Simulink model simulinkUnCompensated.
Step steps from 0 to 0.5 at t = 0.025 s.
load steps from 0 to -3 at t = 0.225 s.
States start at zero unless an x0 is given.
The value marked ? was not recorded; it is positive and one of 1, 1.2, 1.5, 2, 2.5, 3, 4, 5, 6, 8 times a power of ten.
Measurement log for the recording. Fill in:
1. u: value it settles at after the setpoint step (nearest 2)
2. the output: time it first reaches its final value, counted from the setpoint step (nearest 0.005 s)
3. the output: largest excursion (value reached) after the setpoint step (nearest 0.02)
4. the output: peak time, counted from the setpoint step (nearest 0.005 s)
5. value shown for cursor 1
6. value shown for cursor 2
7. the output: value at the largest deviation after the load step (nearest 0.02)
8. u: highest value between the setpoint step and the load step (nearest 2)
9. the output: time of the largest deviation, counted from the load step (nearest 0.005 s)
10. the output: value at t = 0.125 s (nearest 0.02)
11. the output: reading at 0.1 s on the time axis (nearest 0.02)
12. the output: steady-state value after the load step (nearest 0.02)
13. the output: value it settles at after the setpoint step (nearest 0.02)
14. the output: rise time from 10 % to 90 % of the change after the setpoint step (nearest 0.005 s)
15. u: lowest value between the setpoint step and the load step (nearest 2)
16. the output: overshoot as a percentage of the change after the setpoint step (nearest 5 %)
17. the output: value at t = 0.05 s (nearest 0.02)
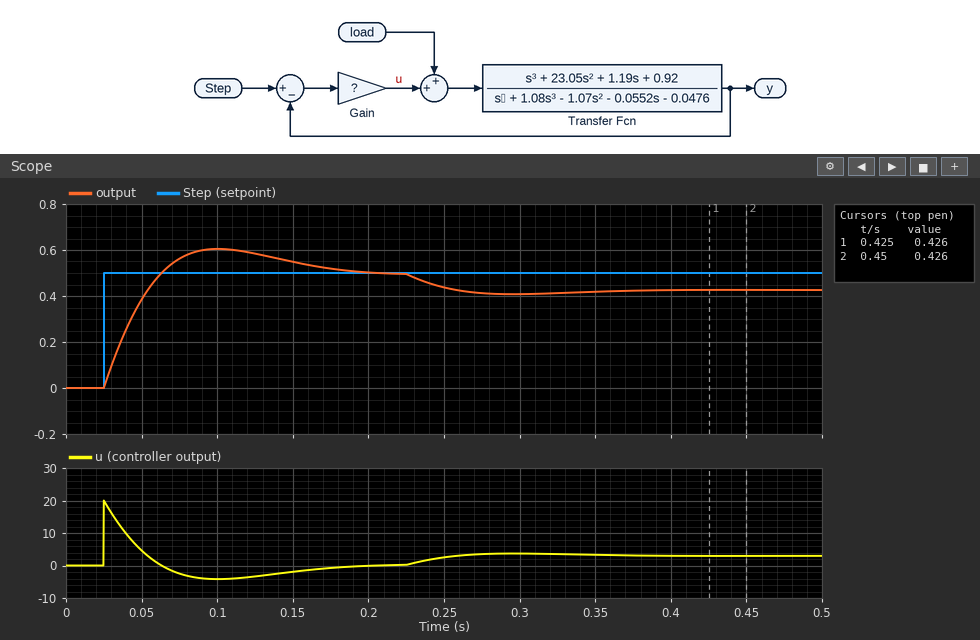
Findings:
0
0.040 s
0.60
0.075 s
0.426
0.426
0.40
20
0.070 s
0.58
0.60
0.42
0.50
0.030 s
-4
20 %
0.38
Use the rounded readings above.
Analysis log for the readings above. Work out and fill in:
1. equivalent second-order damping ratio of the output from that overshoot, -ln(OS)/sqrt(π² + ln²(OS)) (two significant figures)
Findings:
0.46
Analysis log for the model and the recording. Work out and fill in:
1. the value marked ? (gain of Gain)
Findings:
40
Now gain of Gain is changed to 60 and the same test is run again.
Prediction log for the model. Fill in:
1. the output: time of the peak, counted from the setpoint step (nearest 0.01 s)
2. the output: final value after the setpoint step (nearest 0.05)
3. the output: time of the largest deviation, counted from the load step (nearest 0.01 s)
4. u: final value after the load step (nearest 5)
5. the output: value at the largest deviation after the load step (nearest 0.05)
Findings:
0.06 s
0.50
0.06 s
5
0.45
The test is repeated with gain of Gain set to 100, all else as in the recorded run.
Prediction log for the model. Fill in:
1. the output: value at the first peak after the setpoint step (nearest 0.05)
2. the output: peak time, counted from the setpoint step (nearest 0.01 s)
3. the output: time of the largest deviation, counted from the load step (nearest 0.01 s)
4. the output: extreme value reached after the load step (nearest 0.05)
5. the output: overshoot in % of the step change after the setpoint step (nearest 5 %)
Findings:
0.55
0.04 s
0.04 s
0.45
10 %
